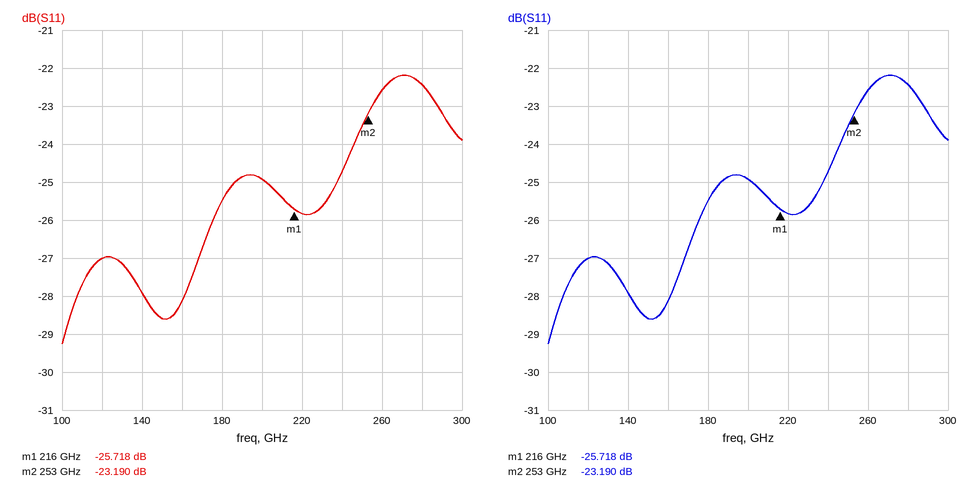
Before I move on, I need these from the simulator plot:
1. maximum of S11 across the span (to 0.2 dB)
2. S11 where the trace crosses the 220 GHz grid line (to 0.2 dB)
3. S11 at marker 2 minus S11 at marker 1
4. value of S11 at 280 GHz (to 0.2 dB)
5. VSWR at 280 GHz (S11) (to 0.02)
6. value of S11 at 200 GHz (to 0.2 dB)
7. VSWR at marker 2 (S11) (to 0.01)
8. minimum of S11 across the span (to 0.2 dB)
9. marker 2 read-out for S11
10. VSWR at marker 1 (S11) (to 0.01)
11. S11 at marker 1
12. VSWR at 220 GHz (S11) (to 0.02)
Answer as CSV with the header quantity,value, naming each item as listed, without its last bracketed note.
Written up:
quantity,value
maximum of S11 across the span,-22.2 dB
S11 where the trace crosses the 220 GHz grid line,-25.8 dB
S11 at marker 2 minus S11 at marker 1,2.528 dB
value of S11 at 280 GHz,-22.4 dB
VSWR at 280 GHz (S11),1.16
value of S11 at 200 GHz,-25.0 dB
VSWR at marker 2 (S11),1.15
minimum of S11 across the span,-29.2 dB
marker 2 read-out for S11,-23.190 dB
VSWR at marker 1 (S11),1.11
S11 at marker 1,-25.718 dB
VSWR at 220 GHz (S11),1.10
